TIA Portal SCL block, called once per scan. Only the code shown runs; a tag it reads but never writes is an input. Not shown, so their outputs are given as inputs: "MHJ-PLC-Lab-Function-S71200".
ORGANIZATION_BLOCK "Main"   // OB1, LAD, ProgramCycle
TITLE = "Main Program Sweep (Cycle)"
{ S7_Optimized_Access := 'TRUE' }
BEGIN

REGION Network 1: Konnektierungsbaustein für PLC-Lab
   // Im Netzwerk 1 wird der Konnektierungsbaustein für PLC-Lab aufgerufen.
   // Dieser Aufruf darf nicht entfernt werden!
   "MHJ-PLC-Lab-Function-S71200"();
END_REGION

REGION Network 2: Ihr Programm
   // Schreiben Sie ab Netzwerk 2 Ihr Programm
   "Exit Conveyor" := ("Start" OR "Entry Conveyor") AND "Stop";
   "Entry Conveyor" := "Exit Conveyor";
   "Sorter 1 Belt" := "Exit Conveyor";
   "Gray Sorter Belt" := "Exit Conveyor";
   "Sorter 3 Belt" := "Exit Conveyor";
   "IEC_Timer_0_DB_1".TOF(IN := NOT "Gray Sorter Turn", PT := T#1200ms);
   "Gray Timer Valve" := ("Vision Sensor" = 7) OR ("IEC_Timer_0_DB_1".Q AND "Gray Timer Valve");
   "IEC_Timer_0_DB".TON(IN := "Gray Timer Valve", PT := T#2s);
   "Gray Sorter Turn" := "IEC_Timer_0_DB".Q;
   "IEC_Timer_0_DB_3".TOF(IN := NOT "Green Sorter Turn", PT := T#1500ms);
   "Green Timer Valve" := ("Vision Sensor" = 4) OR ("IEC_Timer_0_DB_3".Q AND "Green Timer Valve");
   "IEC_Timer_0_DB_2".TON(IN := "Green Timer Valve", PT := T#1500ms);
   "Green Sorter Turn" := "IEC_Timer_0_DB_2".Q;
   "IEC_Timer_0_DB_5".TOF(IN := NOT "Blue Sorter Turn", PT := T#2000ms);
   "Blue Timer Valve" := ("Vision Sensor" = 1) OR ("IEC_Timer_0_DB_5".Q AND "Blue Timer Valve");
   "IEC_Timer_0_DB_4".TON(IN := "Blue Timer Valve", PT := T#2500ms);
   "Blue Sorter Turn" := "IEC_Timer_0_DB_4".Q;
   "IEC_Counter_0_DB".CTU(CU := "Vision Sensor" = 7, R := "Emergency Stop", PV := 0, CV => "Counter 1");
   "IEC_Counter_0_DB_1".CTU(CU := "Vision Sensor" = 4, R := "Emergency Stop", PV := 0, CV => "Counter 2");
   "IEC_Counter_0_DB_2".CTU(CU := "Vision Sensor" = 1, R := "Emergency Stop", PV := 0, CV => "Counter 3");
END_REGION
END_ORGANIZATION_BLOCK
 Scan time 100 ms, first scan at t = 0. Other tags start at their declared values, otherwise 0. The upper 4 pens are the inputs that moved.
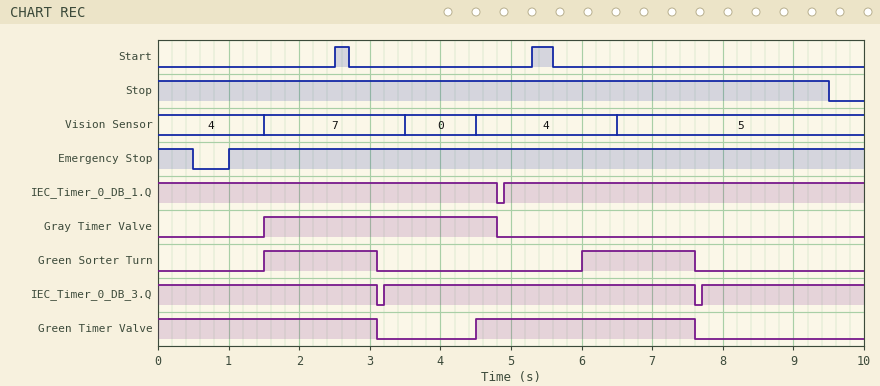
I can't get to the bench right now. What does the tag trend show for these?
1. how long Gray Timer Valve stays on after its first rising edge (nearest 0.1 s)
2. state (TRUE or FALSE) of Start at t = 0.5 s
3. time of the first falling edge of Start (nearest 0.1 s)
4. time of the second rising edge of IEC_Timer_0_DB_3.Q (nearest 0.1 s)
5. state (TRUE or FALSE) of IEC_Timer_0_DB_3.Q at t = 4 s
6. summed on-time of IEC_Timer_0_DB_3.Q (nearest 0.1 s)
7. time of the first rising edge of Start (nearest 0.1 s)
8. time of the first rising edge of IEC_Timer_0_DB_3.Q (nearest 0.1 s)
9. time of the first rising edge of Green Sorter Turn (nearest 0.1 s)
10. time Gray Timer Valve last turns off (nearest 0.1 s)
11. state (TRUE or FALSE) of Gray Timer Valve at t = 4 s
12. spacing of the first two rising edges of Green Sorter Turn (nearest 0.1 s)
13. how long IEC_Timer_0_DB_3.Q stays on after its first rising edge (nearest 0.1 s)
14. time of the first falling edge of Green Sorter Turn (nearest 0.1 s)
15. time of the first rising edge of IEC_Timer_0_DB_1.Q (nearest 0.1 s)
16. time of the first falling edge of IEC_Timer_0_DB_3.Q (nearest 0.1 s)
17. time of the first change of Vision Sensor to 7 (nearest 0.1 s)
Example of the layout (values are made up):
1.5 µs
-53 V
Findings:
3.3 s
FALSE
2.7 s
7.7 s
TRUE
9.8 s
2.5 s
3.2 s
1.5 s
4.8 s
TRUE
4.5 s
4.4 s
3.1 s
4.9 s
3.1 s
1.5 s
